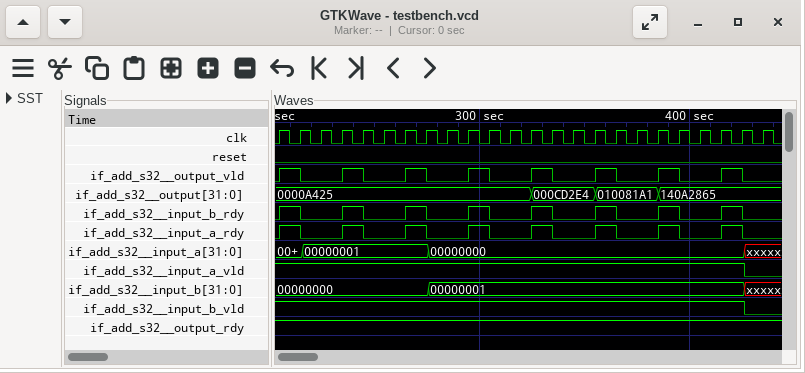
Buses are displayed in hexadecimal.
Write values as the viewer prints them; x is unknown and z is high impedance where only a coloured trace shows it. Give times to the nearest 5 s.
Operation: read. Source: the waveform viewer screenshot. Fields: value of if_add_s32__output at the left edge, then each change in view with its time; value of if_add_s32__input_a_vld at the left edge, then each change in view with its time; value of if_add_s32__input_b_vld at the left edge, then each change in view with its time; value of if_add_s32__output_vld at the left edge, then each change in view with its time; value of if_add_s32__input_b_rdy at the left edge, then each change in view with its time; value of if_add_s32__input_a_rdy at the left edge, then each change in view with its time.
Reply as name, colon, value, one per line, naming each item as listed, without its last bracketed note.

value of if_add_s32__output at the left edge, then each change in view with its time: 0000A425, 000CD2E4 at 325 s, 010081A1 at 355 s, 140A2865 at 385 s
value of if_add_s32__input_a_vld at the left edge, then each change in view with its time: 1, 0 at 425 s
value of if_add_s32__input_b_vld at the left edge, then each change in view with its time: 1, 0 at 425 s
value of if_add_s32__output_vld at the left edge, then each change in view with its time: 0, 1 at 205 s, 0 at 215 s, 1 at 235 s, 0 at 245 s, 1 at 265 s, 0 at 275 s, 1 at 295 s, 0 at 305 s, 1 at 325 s, 0 at 335 s, 1 at 355 s, 0 at 365 s, 1 at 385 s, 0 at 395 s, 1 at 415 s, 0 at 425 s
value of if_add_s32__input_b_rdy at the left edge, then each change in view with its time: 0, 1 at 205 s, 0 at 215 s, 1 at 235 s, 0 at 245 s, 1 at 265 s, 0 at 275 s, 1 at 295 s, 0 at 305 s, 1 at 325 s, 0 at 335 s, 1 at 355 s, 0 at 365 s, 1 at 385 s, 0 at 395 s, 1 at 415 s, 0 at 425 s
value of if_add_s32__input_a_rdy at the left edge, then each change in view with its time: 0, 1 at 205 s, 0 at 215 s, 1 at 235 s, 0 at 245 s, 1 at 265 s, 0 at 275 s, 1 at 295 s, 0 at 305 s, 1 at 325 s, 0 at 335 s, 1 at 355 s, 0 at 365 s, 1 at 385 s, 0 at 395 s, 1 at 415 s, 0 at 425 s
